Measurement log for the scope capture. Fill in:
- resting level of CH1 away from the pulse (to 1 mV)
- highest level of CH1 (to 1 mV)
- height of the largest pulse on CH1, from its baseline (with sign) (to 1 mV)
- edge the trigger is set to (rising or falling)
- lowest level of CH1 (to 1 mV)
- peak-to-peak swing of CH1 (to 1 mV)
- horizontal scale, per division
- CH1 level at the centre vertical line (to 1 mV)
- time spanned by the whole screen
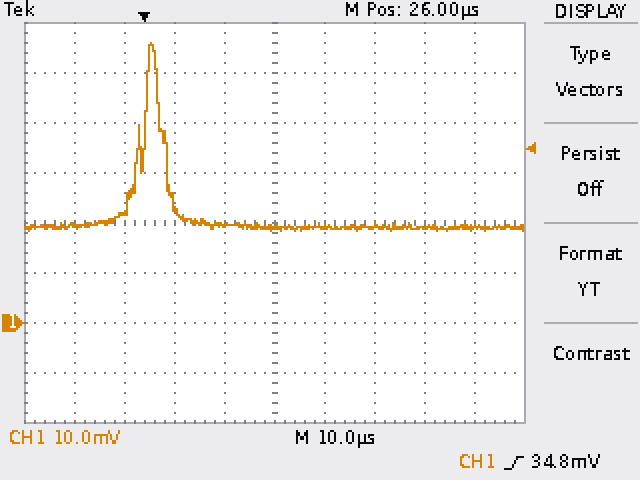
19 mV
56 mV
+37 mV
rising
18 mV
38 mV
10 µs
19 mV
100 µs
